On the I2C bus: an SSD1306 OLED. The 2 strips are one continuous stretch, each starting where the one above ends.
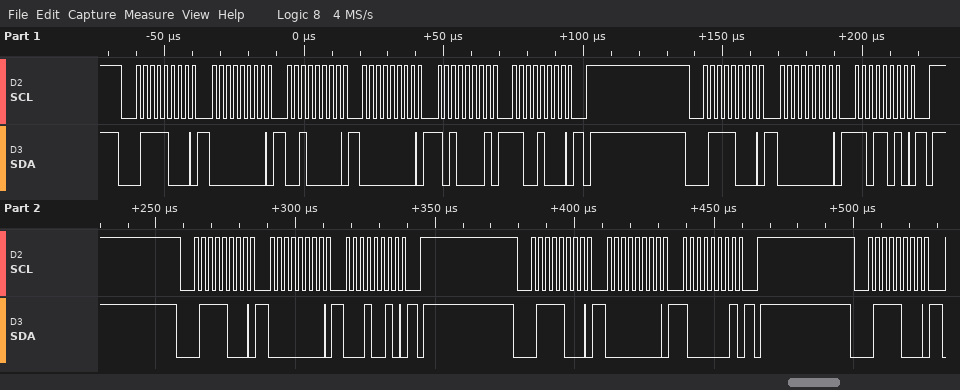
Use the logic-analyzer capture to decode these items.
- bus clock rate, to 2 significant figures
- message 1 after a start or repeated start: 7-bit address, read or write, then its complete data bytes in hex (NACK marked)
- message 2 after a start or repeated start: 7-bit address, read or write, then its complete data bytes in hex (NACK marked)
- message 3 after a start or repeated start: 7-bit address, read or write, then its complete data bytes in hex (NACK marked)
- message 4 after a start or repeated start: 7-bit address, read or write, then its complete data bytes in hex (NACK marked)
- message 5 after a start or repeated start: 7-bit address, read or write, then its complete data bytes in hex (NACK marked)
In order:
400 kHz
0x3C write: 00 20 00 A1 C8
0x3C write: 00 DA
0x3C write: 00 12
0x3C write: 00 81
0x3C write
